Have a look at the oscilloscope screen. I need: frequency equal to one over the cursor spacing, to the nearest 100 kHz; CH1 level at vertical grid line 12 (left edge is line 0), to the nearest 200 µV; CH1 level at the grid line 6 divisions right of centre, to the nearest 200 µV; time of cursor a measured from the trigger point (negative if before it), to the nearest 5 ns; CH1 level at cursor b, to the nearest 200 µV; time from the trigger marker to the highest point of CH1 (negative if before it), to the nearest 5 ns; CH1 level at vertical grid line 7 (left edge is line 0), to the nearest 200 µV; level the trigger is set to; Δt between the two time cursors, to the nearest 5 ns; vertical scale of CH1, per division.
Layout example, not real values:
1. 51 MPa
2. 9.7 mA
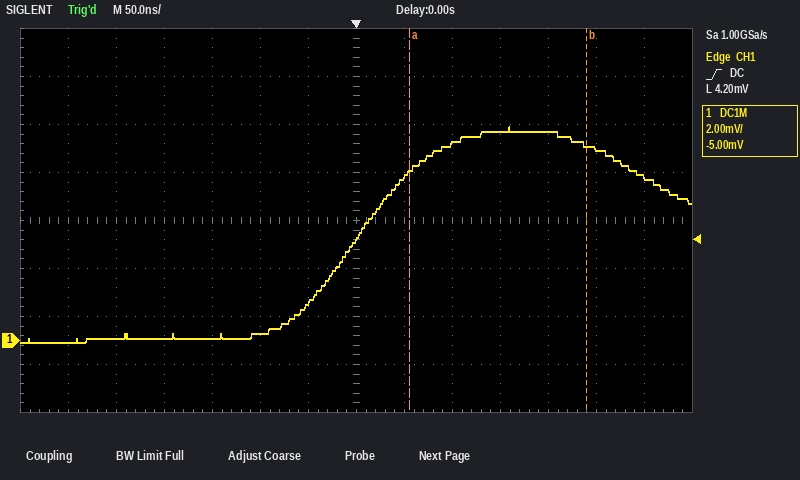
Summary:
1. 5.4 MHz
2. 8.0 mV
3. 6.8 mV
4. +55 ns
5. 8.2 mV
6. +160 ns
7. 4.2 mV
8. 4.20 mV
9. 185 ns
10. 2 mV
